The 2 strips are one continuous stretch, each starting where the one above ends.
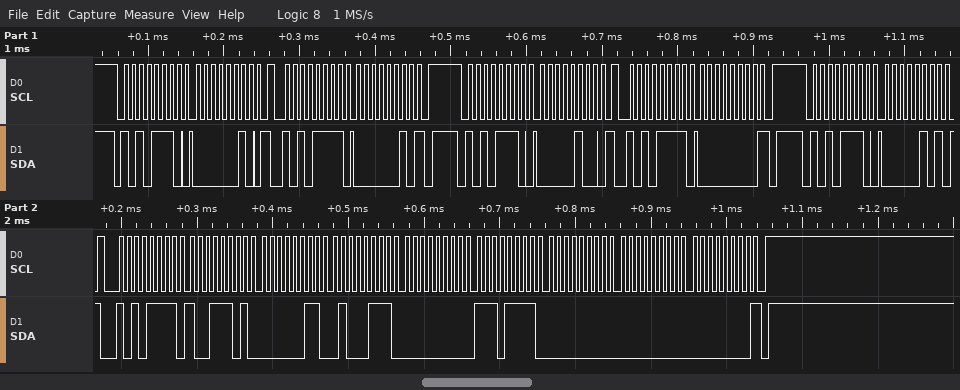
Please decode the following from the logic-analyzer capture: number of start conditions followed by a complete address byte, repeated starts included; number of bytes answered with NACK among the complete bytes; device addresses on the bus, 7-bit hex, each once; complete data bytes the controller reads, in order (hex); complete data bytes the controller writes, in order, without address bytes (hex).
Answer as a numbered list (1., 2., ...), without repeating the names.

1. 6
2. 3
3. 0x57
4. 02 00 9D 03 47 00 EF 00 00 00
5. 02 04 05
